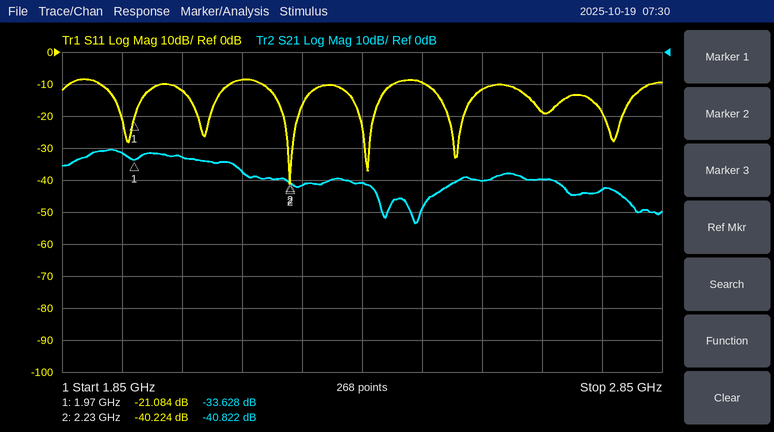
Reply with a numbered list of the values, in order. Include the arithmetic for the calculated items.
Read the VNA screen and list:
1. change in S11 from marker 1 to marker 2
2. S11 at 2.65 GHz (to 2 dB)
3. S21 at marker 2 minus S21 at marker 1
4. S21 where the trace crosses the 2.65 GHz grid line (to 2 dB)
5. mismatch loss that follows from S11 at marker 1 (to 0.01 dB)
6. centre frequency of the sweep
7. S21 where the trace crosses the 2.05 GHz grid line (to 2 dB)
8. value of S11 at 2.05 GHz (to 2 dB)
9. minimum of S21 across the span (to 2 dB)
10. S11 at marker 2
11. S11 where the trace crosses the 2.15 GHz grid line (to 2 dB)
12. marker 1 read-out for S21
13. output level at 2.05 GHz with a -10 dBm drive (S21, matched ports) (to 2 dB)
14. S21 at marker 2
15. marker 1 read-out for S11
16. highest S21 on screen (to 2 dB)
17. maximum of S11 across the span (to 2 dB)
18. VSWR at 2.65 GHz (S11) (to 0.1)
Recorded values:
1. -40.224 − (-21.084) = -19.140 dB
2. -18 dB
3. -40.822 − (-33.628) = -7.194 dB
4. -40 dB
5. −10 log10(1 − 10^(-21.084/10)) ≈ 0.03 dB
6. 2.35 GHz
7. -32 dB
8. -12 dB
9. -54 dB
10. -40.224 dB
11. -8 dB
12. -33.628 dB
13. -10 dBm + (-32 dB) = -42 dBm
14. -40.822 dB
15. -21.084 dB
16. -30 dB
17. -8 dB
18. |Γ| = 10^(-18/20) = 0.1259; VSWR = (1 + 0.1259)/(1 − 0.1259) ≈ 1.3
